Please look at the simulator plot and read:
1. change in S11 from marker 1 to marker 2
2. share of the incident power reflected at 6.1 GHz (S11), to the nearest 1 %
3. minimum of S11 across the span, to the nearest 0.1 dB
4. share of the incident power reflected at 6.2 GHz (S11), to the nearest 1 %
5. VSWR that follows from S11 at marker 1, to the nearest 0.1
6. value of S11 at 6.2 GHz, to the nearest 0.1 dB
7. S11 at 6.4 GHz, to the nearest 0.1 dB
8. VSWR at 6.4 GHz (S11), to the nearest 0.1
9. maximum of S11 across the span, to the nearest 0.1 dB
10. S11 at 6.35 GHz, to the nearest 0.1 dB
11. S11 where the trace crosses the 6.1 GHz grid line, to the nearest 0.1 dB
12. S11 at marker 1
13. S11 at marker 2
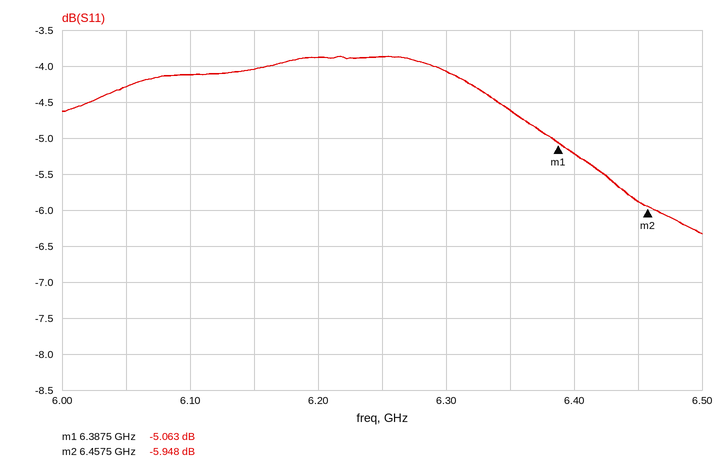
-0.885 dB
39 %
-6.3 dB
41 %
3.5
-3.9 dB
-5.2 dB
3.4
-3.9 dB
-4.6 dB
-4.1 dB
-5.063 dB
-5.948 dB
